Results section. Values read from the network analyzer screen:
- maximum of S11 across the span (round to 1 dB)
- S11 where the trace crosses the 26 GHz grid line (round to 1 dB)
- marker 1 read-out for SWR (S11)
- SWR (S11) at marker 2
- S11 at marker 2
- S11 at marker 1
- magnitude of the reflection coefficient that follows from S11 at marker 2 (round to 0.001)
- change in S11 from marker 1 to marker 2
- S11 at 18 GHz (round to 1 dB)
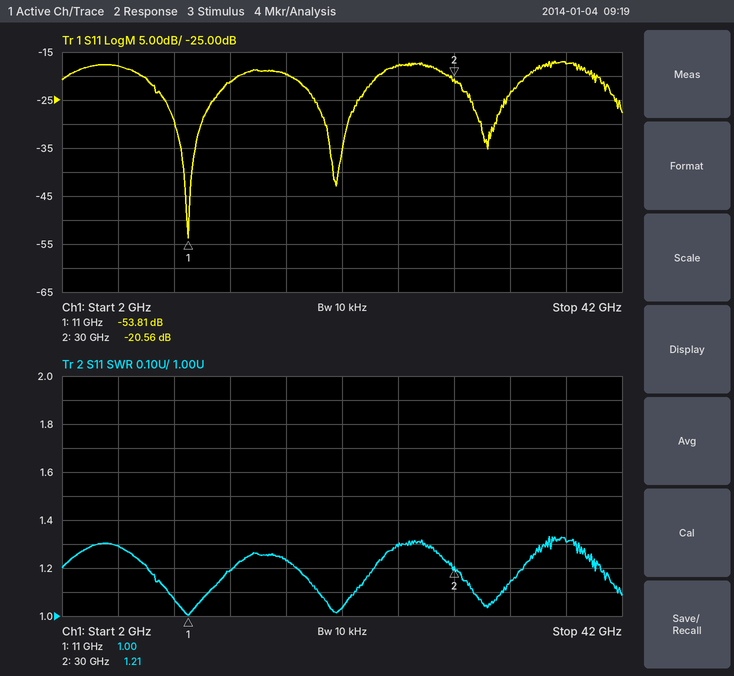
-17 dB
-18 dB
1.00
1.21
-20.56 dB
-53.81 dB
0.094
33.25 dB
-20 dB
